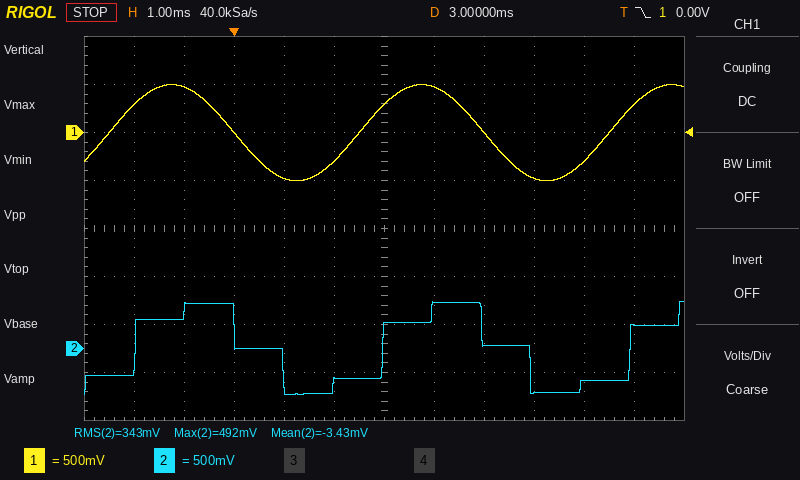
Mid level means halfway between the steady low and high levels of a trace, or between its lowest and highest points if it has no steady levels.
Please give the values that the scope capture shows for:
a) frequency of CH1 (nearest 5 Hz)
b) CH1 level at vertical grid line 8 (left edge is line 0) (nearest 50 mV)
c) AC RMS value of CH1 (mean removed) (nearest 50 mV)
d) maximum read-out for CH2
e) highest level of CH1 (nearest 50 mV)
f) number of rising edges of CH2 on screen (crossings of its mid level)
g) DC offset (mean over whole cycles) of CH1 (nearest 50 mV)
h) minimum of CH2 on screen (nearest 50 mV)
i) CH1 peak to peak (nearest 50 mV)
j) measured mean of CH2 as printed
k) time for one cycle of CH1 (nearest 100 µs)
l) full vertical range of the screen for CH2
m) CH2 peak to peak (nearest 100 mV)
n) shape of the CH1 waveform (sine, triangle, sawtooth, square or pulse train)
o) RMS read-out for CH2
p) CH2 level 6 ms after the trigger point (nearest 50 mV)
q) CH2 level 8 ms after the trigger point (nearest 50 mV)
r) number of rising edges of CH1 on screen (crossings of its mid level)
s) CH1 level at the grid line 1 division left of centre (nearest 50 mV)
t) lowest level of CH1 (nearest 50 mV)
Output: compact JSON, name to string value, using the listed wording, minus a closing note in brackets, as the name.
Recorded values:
{"frequency of CH1": "200 Hz", "CH1 level at vertical grid line 8 (left edge is line 0)": "0 mV", "AC RMS value of CH1 (mean removed)": "350 mV", "maximum read-out for CH2": "492 mV", "highest level of CH1": "500 mV", "number of rising edges of CH2 on screen": "3", "DC offset (mean over whole cycles) of CH1": "0 mV", "minimum of CH2 on screen": "-500 mV", "CH1 peak to peak": "1.00 V", "measured mean of CH2 as printed": "-3.43 mV", "time for one cycle of CH1": "5.0 ms", "full vertical range of the screen for CH2": "4 V", "CH2 peak to peak": "1.00 V", "shape of the CH1 waveform": "sine", "RMS read-out for CH2": "343 mV", "CH2 level 6 ms after the trigger point": "-450 mV", "CH2 level 8 ms after the trigger point": "250 mV", "number of rising edges of CH1 on screen": "3", "CH1 level at the grid line 1 division left of centre": "-300 mV", "lowest level of CH1": "-500 mV"}
